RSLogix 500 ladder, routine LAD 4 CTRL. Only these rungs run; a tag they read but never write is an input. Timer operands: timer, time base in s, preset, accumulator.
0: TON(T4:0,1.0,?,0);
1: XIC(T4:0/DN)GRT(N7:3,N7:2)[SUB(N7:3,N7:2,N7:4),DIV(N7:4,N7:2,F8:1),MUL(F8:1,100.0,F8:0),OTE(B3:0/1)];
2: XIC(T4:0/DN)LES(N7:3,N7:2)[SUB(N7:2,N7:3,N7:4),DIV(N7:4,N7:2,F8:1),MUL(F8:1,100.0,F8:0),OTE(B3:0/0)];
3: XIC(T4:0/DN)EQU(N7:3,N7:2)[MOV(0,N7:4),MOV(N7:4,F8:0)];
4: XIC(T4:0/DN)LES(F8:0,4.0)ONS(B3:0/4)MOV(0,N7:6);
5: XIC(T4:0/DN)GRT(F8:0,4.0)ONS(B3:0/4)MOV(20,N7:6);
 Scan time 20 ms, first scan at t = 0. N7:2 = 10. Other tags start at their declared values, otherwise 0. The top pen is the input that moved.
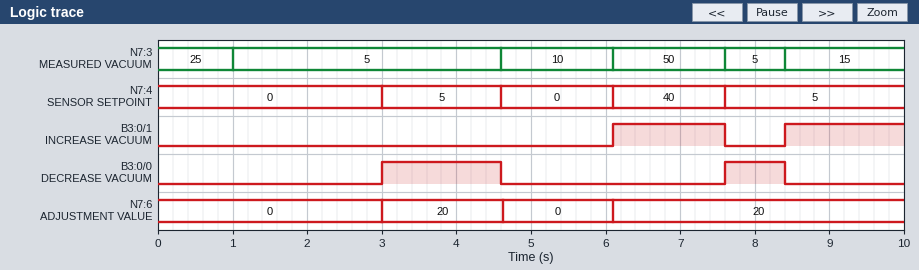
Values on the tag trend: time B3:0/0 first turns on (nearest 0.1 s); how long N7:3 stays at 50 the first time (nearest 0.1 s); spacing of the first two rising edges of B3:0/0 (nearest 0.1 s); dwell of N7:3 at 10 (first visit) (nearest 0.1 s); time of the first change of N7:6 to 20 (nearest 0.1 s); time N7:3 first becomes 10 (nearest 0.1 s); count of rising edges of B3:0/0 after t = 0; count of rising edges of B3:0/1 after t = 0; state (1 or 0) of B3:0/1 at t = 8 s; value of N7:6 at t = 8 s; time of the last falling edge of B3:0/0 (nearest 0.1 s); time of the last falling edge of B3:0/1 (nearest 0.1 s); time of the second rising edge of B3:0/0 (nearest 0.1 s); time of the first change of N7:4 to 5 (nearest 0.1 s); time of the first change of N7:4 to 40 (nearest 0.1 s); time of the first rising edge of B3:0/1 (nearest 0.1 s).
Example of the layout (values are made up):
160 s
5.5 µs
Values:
3.0 s
1.5 s
4.6 s
1.5 s
3.0 s
4.6 s
2
2
0
20
8.4 s
7.6 s
7.6 s
3.0 s
6.1 s
6.1 s
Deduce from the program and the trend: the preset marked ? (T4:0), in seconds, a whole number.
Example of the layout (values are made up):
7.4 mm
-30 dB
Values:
3 s
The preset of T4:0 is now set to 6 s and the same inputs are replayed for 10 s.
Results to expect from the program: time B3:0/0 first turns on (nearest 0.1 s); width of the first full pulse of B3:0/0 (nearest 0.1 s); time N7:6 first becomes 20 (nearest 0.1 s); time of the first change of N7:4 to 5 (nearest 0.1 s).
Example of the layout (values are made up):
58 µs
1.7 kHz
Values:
7.6 s
0.8 s
6.1 s
7.6 s
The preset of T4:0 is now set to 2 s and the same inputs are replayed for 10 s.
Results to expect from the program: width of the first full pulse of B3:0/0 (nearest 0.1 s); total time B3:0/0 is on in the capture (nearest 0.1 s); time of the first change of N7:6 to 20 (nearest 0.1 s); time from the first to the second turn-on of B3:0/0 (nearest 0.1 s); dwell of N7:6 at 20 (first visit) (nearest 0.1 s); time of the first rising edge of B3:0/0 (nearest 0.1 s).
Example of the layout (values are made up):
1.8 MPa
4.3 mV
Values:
2.6 s
3.4 s
2.0 s
5.6 s
2.6 s
2.0 s
